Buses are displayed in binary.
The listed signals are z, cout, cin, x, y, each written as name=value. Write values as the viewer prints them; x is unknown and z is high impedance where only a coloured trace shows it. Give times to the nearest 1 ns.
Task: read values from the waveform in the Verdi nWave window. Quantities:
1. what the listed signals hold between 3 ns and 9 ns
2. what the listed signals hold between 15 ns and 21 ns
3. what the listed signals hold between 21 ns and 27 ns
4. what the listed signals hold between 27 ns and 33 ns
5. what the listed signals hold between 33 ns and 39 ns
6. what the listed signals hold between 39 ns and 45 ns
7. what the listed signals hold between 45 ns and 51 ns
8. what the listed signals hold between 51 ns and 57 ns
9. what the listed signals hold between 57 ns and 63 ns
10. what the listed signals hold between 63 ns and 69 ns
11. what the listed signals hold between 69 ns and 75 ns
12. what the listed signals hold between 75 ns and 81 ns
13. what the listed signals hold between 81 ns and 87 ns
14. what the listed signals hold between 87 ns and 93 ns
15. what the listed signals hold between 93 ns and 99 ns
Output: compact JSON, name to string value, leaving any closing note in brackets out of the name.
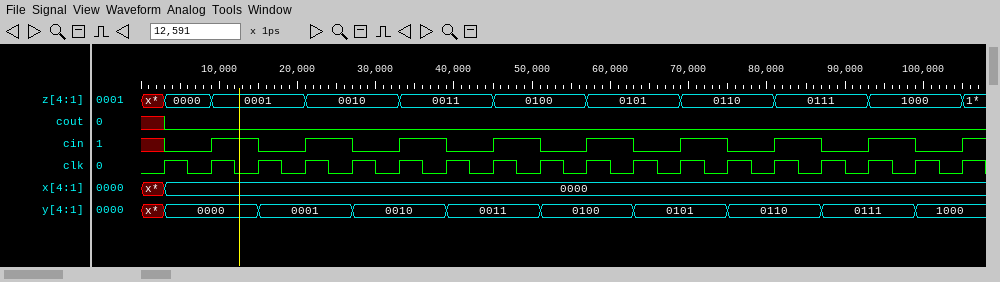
{"what the listed signals hold between 3 ns and 9 ns": "z=0000, cout=0, cin=0, x=0000, y=0000", "what the listed signals hold between 15 ns and 21 ns": "z=0001, cout=0, cin=0, x=0000, y=0001", "what the listed signals hold between 21 ns and 27 ns": "z=0010, cout=0, cin=1, x=0000, y=0001", "what the listed signals hold between 27 ns and 33 ns": "z=0010, cout=0, cin=0, x=0000, y=0010", "what the listed signals hold between 33 ns and 39 ns": "z=0011, cout=0, cin=1, x=0000, y=0010", "what the listed signals hold between 39 ns and 45 ns": "z=0011, cout=0, cin=0, x=0000, y=0011", "what the listed signals hold between 45 ns and 51 ns": "z=0100, cout=0, cin=1, x=0000, y=0011", "what the listed signals hold between 51 ns and 57 ns": "z=0100, cout=0, cin=0, x=0000, y=0100", "what the listed signals hold between 57 ns and 63 ns": "z=0101, cout=0, cin=1, x=0000, y=0100", "what the listed signals hold between 63 ns and 69 ns": "z=0101, cout=0, cin=0, x=0000, y=0101", "what the listed signals hold between 69 ns and 75 ns": "z=0110, cout=0, cin=1, x=0000, y=0101", "what the listed signals hold between 75 ns and 81 ns": "z=0110, cout=0, cin=0, x=0000, y=0110", "what the listed signals hold between 81 ns and 87 ns": "z=0111, cout=0, cin=1, x=0000, y=0110", "what the listed signals hold between 87 ns and 93 ns": "z=0111, cout=0, cin=0, x=0000, y=0111", "what the listed signals hold between 93 ns and 99 ns": "z=1000, cout=0, cin=1, x=0000, y=0111"}
